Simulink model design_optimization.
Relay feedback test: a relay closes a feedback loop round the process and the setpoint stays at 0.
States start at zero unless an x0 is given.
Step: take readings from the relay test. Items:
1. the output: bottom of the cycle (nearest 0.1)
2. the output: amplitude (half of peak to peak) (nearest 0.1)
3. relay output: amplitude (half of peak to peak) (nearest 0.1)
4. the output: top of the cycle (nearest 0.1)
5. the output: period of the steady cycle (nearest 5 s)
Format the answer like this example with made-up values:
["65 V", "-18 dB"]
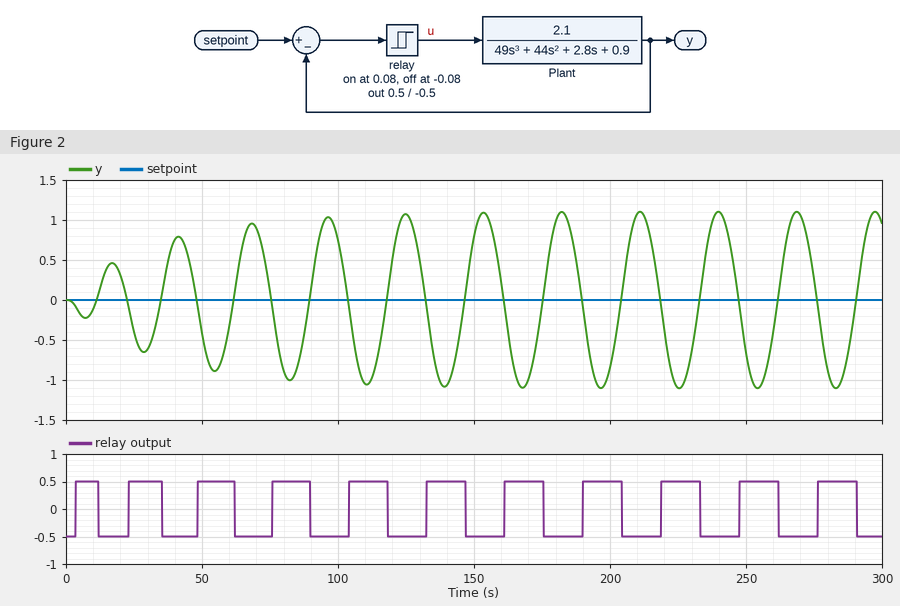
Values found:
["-1.1", "1.1", "0.5", "1.1", "30 s"]
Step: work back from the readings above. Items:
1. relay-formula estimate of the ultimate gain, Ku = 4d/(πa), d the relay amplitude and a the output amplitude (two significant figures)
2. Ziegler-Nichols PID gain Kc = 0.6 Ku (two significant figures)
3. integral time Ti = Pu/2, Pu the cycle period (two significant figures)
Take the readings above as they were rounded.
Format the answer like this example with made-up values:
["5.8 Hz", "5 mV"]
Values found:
["0.58", "0.35", "15 s"]
